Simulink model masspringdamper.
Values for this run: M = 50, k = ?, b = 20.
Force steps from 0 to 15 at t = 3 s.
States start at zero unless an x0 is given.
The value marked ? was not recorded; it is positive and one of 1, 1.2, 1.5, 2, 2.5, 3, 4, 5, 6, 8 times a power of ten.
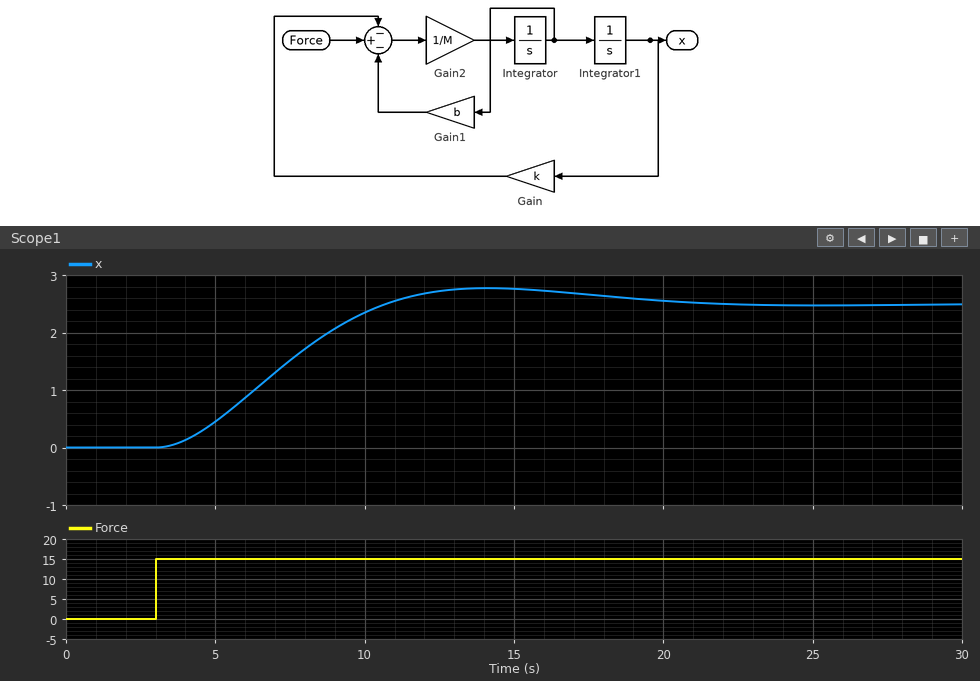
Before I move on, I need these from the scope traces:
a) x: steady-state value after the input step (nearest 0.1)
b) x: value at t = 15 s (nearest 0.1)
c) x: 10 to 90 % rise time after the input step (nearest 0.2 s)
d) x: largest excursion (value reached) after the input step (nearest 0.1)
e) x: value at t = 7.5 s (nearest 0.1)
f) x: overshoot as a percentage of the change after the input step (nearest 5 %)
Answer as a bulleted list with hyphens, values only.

- 2.5
- 2.8
- 5.2 s
- 2.8
- 1.5
- 10 %
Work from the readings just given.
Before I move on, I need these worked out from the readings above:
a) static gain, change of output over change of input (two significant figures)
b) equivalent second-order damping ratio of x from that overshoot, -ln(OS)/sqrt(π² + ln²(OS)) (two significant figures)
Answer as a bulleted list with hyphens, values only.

- 0.17
- 0.59
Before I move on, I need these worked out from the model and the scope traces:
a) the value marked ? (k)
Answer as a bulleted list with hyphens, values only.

- 6
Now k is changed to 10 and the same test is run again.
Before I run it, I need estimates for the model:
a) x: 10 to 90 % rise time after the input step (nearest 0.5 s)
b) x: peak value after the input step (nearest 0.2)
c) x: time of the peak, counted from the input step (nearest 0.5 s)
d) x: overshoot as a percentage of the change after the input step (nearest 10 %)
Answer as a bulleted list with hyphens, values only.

- 3.5 s
- 1.8
- 8.0 s
- 20 %
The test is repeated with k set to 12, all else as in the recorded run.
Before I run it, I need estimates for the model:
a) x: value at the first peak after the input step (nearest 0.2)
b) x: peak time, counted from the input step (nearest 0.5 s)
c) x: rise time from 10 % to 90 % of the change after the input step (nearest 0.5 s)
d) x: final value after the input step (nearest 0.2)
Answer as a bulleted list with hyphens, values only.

- 1.6
- 7.0 s
- 3.0 s
- 1.2
